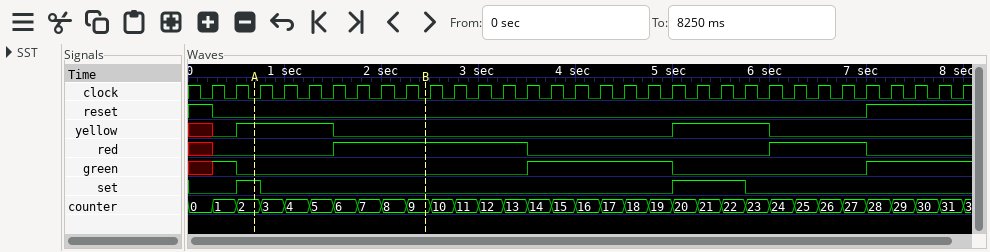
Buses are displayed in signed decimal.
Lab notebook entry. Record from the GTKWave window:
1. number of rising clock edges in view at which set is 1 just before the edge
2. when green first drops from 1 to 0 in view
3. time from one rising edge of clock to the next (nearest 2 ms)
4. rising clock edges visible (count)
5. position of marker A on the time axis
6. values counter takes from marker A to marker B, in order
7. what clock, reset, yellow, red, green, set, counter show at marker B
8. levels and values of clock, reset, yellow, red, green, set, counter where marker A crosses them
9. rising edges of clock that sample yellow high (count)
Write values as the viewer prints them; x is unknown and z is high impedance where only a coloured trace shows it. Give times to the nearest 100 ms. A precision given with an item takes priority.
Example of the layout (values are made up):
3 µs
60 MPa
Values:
4
500 ms
250 ms
32
700 ms
2, 3, 4, 5, 6, 7, 8, 9
clock=0, reset=0, yellow=0, red=1, green=0, set=0, counter=9
clock=0, reset=0, yellow=1, red=0, green=0, set=1, counter=2
8
